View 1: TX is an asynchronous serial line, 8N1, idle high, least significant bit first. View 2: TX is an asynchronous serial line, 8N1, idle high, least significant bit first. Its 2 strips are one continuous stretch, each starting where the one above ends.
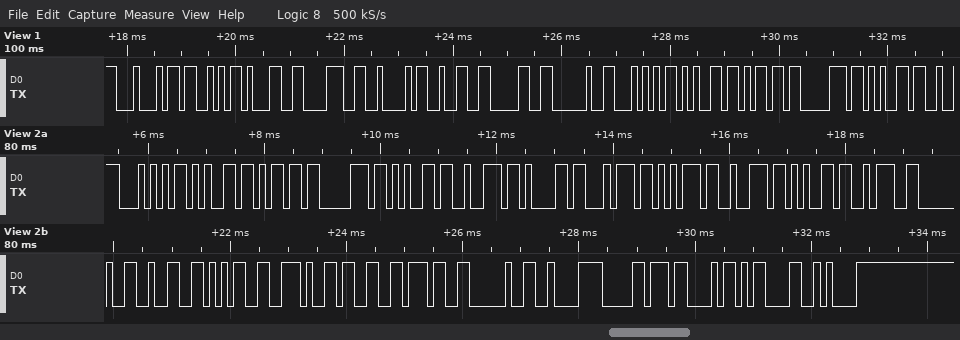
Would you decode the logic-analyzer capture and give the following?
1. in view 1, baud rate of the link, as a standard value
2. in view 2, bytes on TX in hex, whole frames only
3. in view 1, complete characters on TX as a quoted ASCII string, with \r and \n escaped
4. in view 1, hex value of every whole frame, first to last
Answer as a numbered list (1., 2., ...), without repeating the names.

1. 9600 baud
2. 0x54 0x65 0x6D 0x70 0x65 0x72 0x61 0x74 0x75 0x72 0x65 0x3A 0x20 0x32 0x35 0x2E 0x33 0x37 0x20 0xC2 0xB0 0x43 0x0D 0x0A
3. "DS18B20 Tempe"
4. 44 53 31 38 42 32 30 20 54 65 6D 70 65
